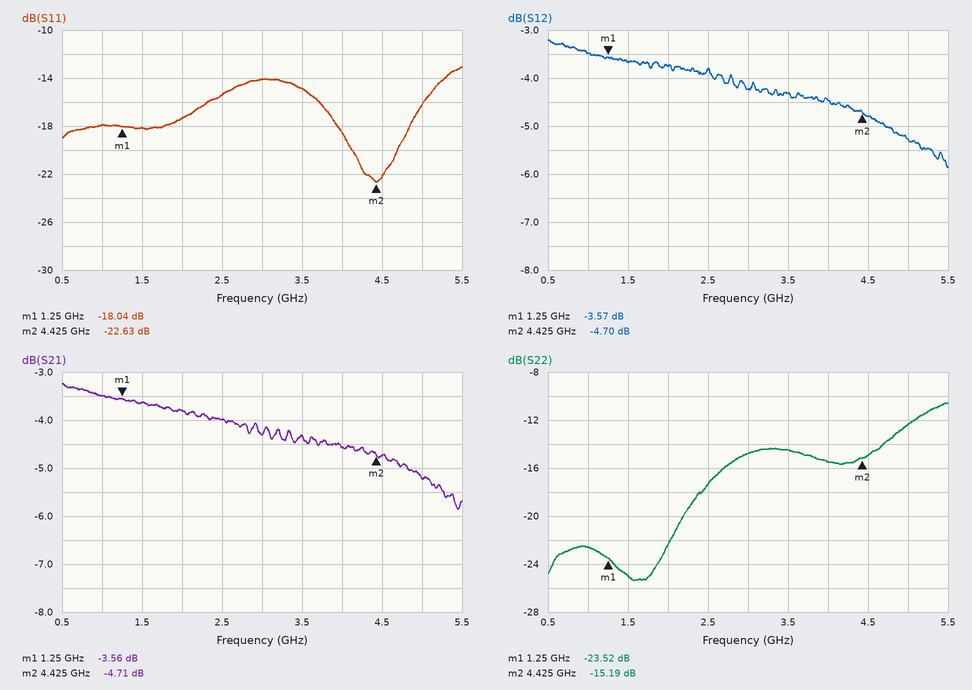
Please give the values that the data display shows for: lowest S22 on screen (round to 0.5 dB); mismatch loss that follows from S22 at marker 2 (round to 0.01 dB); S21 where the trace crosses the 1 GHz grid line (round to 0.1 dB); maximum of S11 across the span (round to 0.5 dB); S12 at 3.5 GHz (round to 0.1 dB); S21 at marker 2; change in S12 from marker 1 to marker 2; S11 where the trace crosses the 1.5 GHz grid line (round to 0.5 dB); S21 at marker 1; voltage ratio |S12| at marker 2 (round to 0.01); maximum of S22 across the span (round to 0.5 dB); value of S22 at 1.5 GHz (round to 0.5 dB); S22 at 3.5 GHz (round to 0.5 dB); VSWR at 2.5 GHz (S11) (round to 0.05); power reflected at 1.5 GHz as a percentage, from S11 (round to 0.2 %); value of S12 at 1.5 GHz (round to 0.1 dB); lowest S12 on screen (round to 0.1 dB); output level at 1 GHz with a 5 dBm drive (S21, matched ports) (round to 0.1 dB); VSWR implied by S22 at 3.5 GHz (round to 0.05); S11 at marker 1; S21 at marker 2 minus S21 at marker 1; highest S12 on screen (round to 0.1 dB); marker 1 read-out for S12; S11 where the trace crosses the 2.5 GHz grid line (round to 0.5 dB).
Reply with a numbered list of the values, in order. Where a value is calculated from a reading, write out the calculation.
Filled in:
1. -25.5 dB
2. −10 log10(1 − 10^(-15.19/10)) ≈ 0.13 dB
3. -3.5 dB
4. -13.0 dB
5. -4.3 dB
6. -4.71 dB
7. -4.7 − (-3.57) = -1.13 dB
8. -18.0 dB
9. -3.56 dB
10. 10^(-4.7/20) ≈ 0.58
11. -10.5 dB
12. -25.0 dB
13. -14.5 dB
14. |Γ| = 10^(-15.5/20) = 0.1679; VSWR = (1 + 0.1679)/(1 − 0.1679) ≈ 1.40
15. 10^(-18/10) ≈ 1.6 %
16. -3.7 dB
17. -5.9 dB
18. 5 dBm + (-3.5 dB) = 1.5 dBm
19. |Γ| = 10^(-14.5/20) = 0.1884; VSWR = (1 + 0.1884)/(1 − 0.1884) ≈ 1.46, so 1.45 to the nearest 0.05
20. -18.04 dB
21. -4.71 − (-3.56) = -1.15 dB
22. -3.2 dB
23. -3.57 dB
24. -15.5 dB
